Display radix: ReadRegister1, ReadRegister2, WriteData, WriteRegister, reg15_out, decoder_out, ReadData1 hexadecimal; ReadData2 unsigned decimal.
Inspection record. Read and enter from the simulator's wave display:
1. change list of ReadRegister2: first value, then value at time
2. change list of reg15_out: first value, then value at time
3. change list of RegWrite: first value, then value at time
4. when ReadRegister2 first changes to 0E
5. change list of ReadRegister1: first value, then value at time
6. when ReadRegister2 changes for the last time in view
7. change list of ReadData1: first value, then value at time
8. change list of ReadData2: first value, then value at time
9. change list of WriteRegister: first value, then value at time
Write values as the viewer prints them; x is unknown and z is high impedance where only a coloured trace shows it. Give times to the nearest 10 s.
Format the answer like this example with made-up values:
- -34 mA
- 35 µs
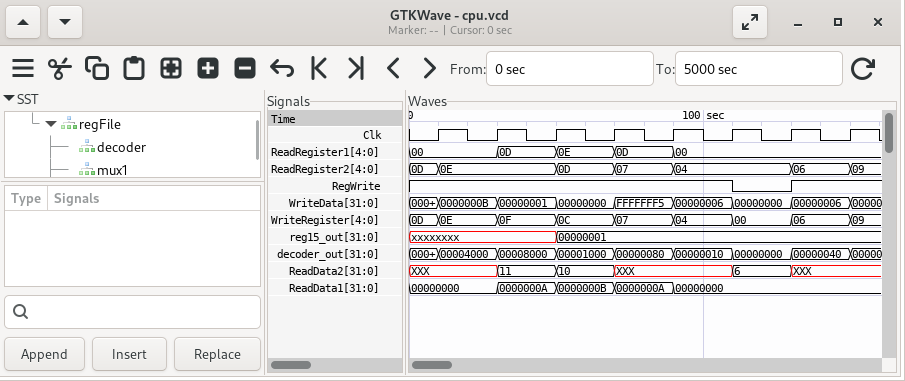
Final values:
- 0D, 0E at 10 s, 0D at 50 s, 07 at 70 s, 04 at 90 s, 06 at 130 s, 09 at 150 s
- xxxxxxxx, 00000001 at 50 s
- 1, 0 at 110 s, 1 at 130 s
- 10 s
- 00, 0D at 30 s, 0E at 50 s, 0D at 70 s, 00 at 90 s
- 150 s
- 00000000, 0000000A at 30 s, 0000000B at 50 s, 0000000A at 70 s, 00000000 at 90 s
- XXX, 11 at 30 s, 10 at 50 s, XXX at 70 s, 6 at 110 s, XXX at 130 s
- 0D, 0E at 10 s, 0F at 30 s, 0C at 50 s, 07 at 70 s, 04 at 90 s, 00 at 110 s, 06 at 130 s, 09 at 150 s
